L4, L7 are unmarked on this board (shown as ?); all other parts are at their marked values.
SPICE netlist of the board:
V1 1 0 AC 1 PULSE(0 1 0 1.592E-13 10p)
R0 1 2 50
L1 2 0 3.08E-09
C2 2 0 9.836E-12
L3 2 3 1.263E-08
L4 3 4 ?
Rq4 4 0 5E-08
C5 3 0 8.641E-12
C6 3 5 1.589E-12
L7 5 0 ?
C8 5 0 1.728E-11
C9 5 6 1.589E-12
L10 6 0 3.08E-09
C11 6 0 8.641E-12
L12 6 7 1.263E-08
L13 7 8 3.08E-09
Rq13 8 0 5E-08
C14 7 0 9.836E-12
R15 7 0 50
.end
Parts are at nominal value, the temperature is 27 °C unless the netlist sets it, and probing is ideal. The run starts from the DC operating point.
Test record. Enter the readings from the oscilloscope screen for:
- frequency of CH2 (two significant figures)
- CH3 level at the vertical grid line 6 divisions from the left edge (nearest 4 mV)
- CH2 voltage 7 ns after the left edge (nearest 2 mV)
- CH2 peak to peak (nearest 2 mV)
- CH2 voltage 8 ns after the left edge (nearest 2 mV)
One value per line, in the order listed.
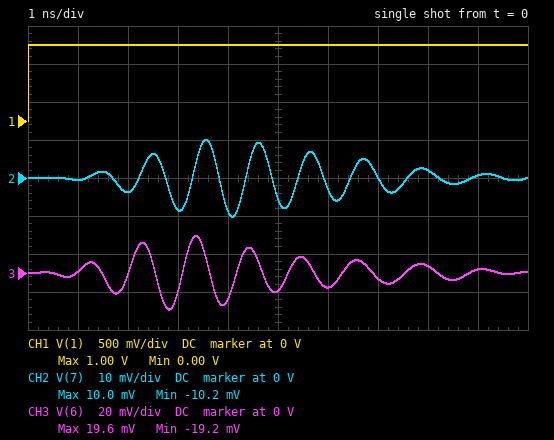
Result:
950 MHz
-8 mV
0 V
20 mV
2 mV
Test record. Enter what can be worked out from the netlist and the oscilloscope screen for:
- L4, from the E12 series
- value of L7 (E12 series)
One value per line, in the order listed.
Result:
3.9 nH
2.7 nH
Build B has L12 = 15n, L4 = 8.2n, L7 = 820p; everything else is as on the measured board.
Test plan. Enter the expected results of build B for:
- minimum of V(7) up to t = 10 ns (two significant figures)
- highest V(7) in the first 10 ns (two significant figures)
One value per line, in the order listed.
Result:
-3.6 mV
3.5 mV
